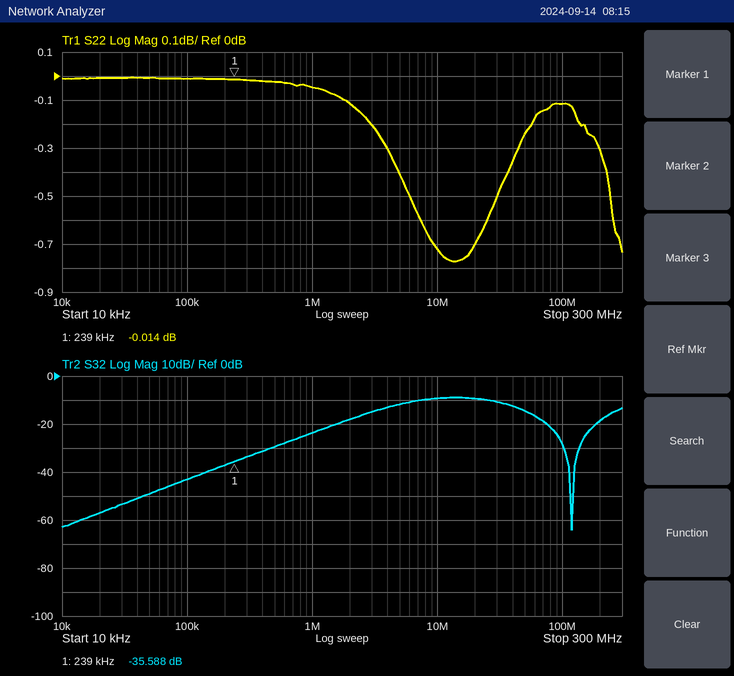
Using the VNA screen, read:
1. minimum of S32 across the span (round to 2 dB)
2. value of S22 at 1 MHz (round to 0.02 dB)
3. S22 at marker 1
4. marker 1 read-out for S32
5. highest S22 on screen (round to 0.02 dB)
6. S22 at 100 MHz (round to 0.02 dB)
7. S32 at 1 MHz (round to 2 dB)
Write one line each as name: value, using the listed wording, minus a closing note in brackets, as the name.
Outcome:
minimum of S32 across the span: -64 dB
value of S22 at 1 MHz: -0.04 dB
S22 at marker 1: -0.014 dB
marker 1 read-out for S32: -35.588 dB
highest S22 on screen: 0.00 dB
S22 at 100 MHz: -0.12 dB
S32 at 1 MHz: -24 dB
